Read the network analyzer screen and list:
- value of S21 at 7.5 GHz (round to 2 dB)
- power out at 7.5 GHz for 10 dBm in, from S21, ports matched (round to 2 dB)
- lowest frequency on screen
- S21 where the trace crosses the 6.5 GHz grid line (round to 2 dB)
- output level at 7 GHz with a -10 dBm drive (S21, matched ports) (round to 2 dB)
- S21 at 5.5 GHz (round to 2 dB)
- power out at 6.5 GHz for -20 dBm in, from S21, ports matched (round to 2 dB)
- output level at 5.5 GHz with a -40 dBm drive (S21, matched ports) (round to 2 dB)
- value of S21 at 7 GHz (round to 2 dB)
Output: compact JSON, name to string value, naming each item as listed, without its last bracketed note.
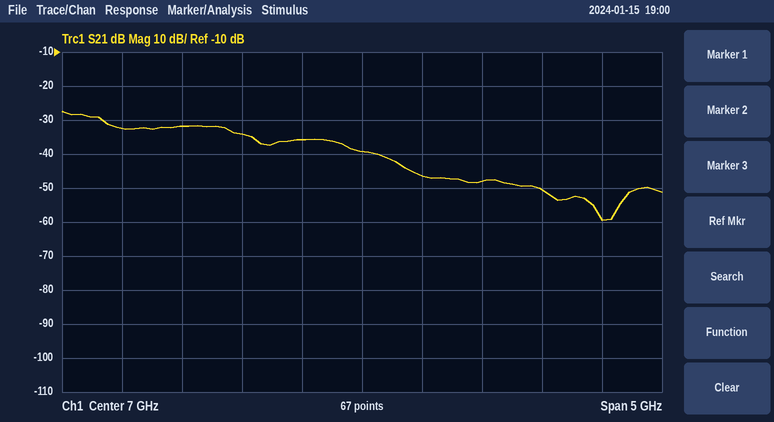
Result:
{"value of S21 at 7.5 GHz": "-46 dB", "power out at 7.5 GHz for 10 dBm in, from S21, ports matched": "-36 dBm", "lowest frequency on screen": "4.5 GHz", "S21 where the trace crosses the 6.5 GHz grid line": "-36 dB", "output level at 7 GHz with a -10 dBm drive (S21, matched ports)": "-50 dBm", "S21 at 5.5 GHz": "-32 dB", "power out at 6.5 GHz for -20 dBm in, from S21, ports matched": "-56 dBm", "output level at 5.5 GHz with a -40 dBm drive (S21, matched ports)": "-72 dBm", "value of S21 at 7 GHz": "-40 dB"}
